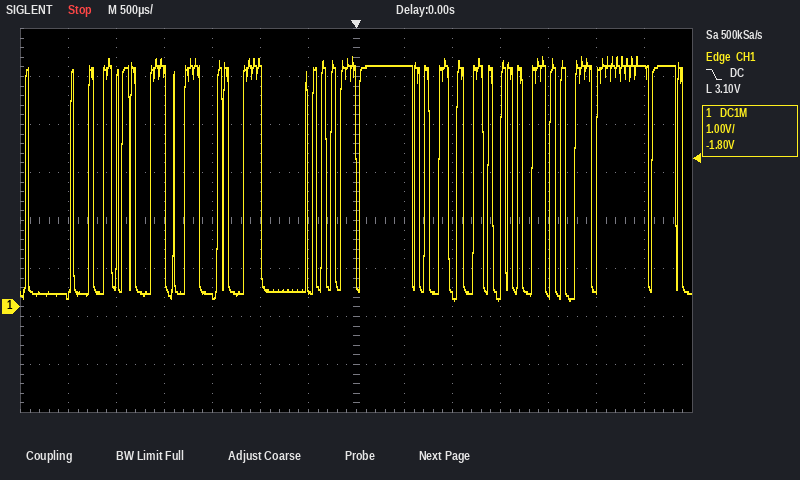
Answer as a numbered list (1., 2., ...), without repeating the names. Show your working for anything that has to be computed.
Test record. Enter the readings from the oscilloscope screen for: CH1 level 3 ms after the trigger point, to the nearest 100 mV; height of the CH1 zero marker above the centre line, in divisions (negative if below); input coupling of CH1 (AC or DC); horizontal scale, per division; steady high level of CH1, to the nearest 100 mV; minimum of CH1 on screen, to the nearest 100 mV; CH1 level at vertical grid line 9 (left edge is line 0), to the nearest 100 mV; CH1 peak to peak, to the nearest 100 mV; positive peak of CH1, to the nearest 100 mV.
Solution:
1. 5.0 V
2. -1.8 div
3. DC
4. 500 µs
5. 5.0 V
6. 100 mV
7. 300 mV
8. 5.2 V − (100 mV) = 5.1 V
9. 5.2 V
